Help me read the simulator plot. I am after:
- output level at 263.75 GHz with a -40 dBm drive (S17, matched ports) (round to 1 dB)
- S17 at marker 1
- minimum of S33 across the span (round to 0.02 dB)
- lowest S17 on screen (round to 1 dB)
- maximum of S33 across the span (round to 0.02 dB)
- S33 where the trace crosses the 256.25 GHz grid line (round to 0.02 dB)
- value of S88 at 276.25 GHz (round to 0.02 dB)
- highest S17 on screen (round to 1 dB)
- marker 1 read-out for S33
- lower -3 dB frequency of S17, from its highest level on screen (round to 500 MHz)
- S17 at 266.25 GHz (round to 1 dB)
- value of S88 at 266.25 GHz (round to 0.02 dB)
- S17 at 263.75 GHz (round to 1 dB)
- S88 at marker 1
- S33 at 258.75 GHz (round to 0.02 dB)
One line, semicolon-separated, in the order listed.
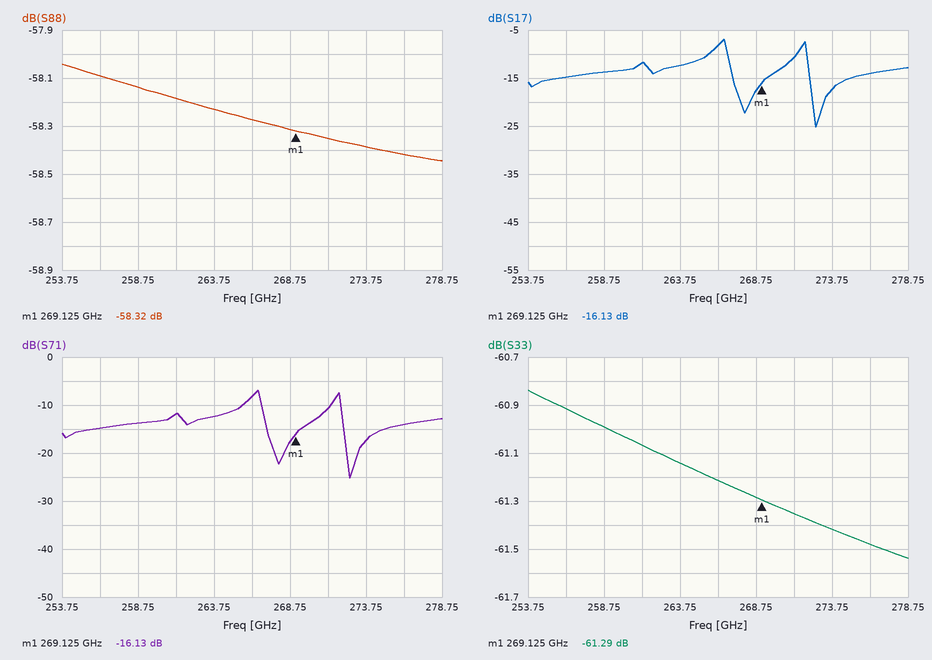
-52 dBm; -16.13 dB; -61.54 dB; -25 dB; -60.84 dB; -60.92 dB; -58.42 dB; -7 dB; -61.29 dB; 265.5 GHz; -8 dB; -58.28 dB; -12 dB; -58.32 dB; -61.00 dB
